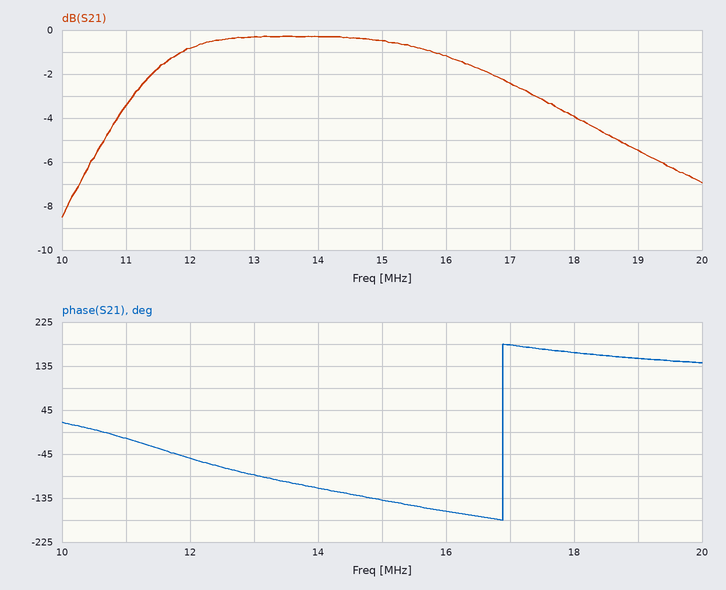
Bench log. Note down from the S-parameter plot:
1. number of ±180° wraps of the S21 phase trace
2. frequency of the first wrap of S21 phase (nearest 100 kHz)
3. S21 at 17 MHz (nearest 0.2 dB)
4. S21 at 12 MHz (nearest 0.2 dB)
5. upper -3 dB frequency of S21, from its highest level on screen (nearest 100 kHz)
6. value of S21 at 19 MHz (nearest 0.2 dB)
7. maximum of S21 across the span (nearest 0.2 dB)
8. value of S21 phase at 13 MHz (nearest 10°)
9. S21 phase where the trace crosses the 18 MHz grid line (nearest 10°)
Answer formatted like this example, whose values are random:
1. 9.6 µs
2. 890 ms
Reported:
1. 1
2. 16.9 MHz
3. -2.4 dB
4. -0.8 dB
5. 17.6 MHz
6. -5.4 dB
7. -0.2 dB
8. -90°
9. 160°
